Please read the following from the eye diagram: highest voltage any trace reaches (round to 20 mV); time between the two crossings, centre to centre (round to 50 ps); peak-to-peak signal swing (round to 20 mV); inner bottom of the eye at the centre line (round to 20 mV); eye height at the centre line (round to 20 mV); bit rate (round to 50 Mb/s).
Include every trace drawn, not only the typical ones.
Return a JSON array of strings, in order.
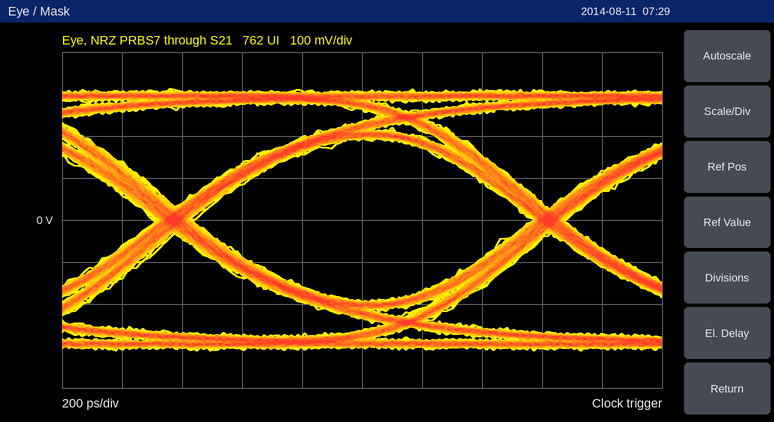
["320 mV", "1.25 ns", "620 mV", "-200 mV", "380 mV", "800 Mb/s"]
